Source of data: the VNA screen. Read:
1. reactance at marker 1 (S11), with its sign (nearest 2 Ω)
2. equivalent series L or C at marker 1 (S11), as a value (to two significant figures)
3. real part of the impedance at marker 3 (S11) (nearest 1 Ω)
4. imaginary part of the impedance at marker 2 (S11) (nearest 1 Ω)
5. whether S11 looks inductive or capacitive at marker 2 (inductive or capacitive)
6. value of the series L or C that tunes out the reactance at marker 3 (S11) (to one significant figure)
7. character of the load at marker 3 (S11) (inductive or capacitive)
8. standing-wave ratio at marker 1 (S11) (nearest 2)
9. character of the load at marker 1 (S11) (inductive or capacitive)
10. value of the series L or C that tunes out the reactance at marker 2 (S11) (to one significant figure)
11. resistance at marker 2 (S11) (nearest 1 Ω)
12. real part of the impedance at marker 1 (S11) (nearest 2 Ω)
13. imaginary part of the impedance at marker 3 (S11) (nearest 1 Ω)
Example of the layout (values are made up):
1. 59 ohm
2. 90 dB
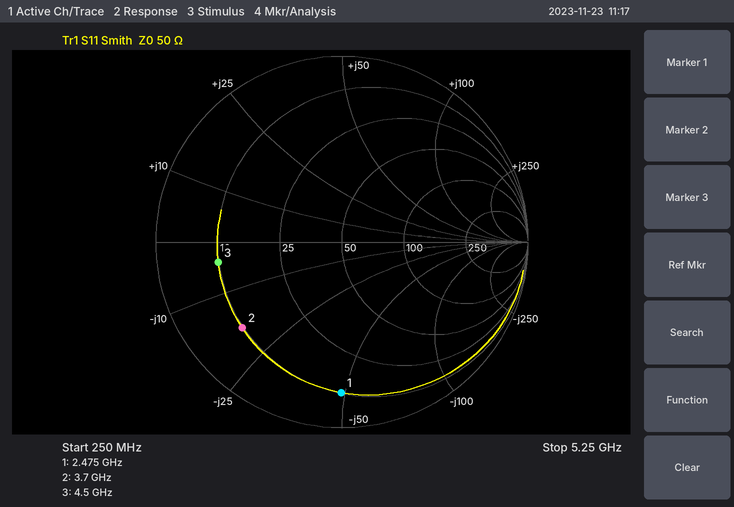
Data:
1. -48 Ω
2. 1.3 pF
3. 10 Ω
4. -18 Ω
5. capacitive
6. 100 pH
7. capacitive
8. 10
9. capacitive
10. 800 pH
11. 10 Ω
12. 10 Ω
13. -4 Ω
